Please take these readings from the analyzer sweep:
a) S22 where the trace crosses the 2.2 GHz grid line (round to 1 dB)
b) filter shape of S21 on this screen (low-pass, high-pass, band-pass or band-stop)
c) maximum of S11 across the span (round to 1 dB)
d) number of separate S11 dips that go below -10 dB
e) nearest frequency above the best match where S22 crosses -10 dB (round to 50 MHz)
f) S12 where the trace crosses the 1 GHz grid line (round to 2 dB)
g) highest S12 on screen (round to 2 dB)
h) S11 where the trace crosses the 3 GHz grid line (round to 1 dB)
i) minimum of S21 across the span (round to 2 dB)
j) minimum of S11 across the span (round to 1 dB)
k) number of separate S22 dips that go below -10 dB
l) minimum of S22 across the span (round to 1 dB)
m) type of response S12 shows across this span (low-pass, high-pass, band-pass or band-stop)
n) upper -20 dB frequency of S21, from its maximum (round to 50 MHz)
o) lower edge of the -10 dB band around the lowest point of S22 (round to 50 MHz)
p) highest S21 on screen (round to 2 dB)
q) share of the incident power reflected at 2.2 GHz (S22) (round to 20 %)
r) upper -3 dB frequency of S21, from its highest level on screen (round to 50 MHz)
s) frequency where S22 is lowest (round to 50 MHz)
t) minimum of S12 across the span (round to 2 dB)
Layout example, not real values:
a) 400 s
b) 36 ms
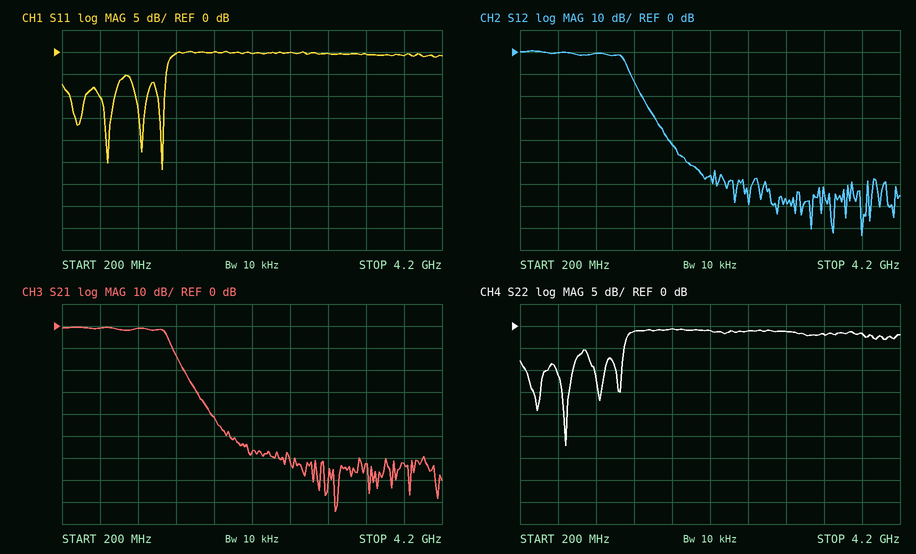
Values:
a) -1 dB
b) low-pass
c) 0 dB
d) 4
e) 750 MHz
f) 0 dB
g) 0 dB
h) 0 dB
i) -84 dB
j) -27 dB
k) 4
l) -27 dB
m) low-pass
n) 1.50 GHz
o) 600 MHz
p) 0 dB
q) 80 %
r) 1.30 GHz
s) 700 MHz
t) -84 dB
